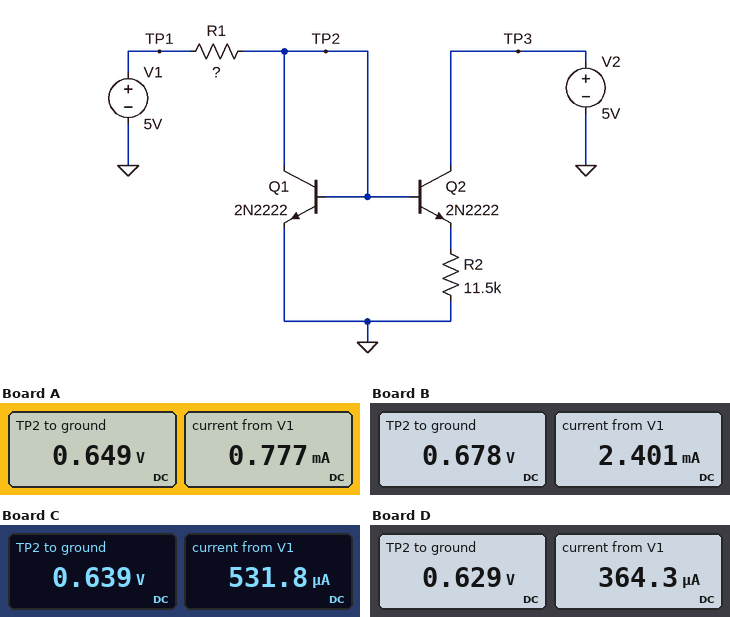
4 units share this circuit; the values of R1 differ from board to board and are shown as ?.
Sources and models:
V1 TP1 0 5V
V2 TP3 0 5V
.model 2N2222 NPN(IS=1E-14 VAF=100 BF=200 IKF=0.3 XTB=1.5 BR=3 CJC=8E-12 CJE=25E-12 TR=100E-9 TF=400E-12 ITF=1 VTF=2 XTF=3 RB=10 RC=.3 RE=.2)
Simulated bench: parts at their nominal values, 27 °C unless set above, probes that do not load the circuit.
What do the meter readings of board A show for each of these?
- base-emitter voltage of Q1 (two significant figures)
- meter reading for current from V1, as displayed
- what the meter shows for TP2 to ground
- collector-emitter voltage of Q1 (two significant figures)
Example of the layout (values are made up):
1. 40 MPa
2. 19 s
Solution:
1. 650 mV
2. 0.777 mA
3. 0.649 V
4. 650 mV
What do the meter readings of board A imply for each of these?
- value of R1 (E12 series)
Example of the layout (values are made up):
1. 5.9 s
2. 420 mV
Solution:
1. 5.6 kΩ
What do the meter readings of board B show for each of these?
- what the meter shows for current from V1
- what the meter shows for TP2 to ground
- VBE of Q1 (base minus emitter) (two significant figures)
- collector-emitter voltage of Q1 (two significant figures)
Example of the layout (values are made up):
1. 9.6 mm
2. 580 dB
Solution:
1. 2.401 mA
2. 0.678 V
3. 680 mV
4. 680 mV
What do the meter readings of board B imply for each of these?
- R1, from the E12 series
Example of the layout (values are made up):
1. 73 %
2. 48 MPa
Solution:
1. 1.8 kΩ
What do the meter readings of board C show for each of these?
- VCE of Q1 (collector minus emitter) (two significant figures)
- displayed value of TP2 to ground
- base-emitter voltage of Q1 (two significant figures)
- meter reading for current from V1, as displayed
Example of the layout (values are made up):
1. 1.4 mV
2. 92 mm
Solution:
1. 640 mV
2. 0.639 V
3. 640 mV
4. 531.8 µA
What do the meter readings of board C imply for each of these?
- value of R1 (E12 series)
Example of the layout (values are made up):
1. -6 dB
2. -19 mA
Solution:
1. 8.2 kΩ
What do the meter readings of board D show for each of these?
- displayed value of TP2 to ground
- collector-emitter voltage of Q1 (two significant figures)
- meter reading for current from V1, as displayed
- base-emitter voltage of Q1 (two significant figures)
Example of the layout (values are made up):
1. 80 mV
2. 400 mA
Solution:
1. 0.629 V
2. 630 mV
3. 364.3 µA
4. 630 mV
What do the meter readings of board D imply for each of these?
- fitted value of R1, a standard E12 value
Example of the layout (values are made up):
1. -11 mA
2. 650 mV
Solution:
1. 12 kΩ
